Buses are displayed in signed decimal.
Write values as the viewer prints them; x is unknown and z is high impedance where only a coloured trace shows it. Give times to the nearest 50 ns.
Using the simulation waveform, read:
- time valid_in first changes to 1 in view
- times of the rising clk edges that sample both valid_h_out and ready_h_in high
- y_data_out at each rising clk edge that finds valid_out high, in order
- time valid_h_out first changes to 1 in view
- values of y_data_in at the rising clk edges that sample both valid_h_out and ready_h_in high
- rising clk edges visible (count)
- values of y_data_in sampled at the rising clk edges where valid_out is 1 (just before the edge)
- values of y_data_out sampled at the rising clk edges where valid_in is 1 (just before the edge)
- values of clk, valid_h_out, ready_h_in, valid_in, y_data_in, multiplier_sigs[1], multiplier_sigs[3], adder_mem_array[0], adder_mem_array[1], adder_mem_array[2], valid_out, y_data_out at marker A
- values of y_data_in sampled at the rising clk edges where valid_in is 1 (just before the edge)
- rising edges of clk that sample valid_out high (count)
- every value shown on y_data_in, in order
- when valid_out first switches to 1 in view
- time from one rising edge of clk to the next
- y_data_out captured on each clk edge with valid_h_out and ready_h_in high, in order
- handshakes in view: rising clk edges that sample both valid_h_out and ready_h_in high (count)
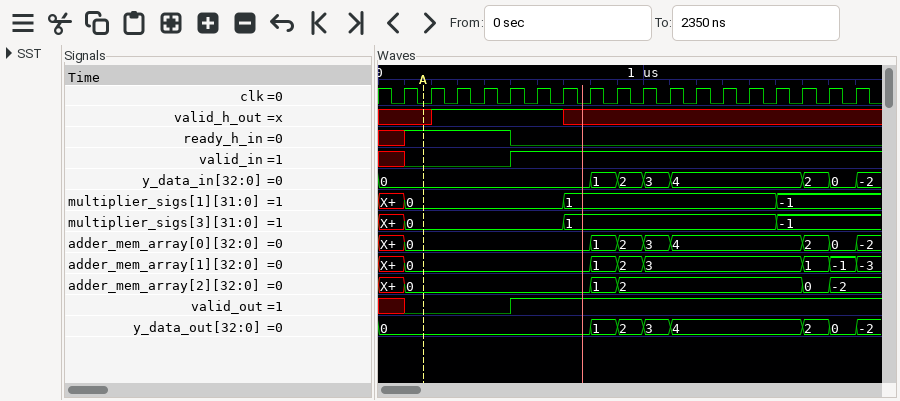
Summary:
500 ns
300 ns, 400 ns, 500 ns
0, 0, 0, 1, 2, 3, 4, 4, 4, 4, 4, 2, 0
200 ns
0, 0, 0
18
0, 0, 0, 1, 2, 3, 4, 4, 4, 4, 4, 2, 0
0, 0, 0, 1, 2, 3, 4, 4, 4, 4, 4, 2, 0
clk=0, valid_h_out=x, ready_h_in=1, valid_in=0, y_data_in=0, multiplier_sigs[1]=0, multiplier_sigs[3]=0, adder_mem_array[0]=0, adder_mem_array[1]=0, adder_mem_array[2]=0, valid_out=0, y_data_out=0
0, 0, 0, 1, 2, 3, 4, 4, 4, 4, 4, 2, 0
13
0, 1, 2, 3, 4, 2, 0, -2
500 ns
100 ns
0, 0, 0
3
